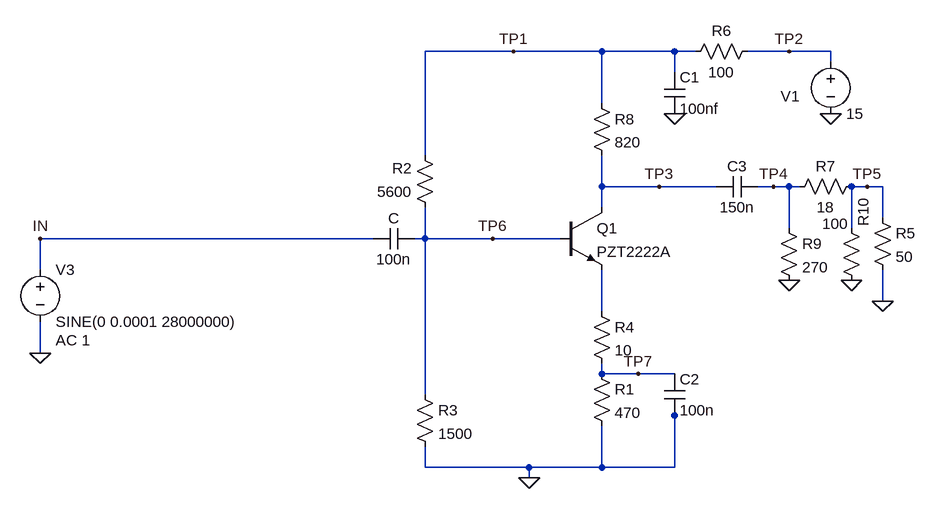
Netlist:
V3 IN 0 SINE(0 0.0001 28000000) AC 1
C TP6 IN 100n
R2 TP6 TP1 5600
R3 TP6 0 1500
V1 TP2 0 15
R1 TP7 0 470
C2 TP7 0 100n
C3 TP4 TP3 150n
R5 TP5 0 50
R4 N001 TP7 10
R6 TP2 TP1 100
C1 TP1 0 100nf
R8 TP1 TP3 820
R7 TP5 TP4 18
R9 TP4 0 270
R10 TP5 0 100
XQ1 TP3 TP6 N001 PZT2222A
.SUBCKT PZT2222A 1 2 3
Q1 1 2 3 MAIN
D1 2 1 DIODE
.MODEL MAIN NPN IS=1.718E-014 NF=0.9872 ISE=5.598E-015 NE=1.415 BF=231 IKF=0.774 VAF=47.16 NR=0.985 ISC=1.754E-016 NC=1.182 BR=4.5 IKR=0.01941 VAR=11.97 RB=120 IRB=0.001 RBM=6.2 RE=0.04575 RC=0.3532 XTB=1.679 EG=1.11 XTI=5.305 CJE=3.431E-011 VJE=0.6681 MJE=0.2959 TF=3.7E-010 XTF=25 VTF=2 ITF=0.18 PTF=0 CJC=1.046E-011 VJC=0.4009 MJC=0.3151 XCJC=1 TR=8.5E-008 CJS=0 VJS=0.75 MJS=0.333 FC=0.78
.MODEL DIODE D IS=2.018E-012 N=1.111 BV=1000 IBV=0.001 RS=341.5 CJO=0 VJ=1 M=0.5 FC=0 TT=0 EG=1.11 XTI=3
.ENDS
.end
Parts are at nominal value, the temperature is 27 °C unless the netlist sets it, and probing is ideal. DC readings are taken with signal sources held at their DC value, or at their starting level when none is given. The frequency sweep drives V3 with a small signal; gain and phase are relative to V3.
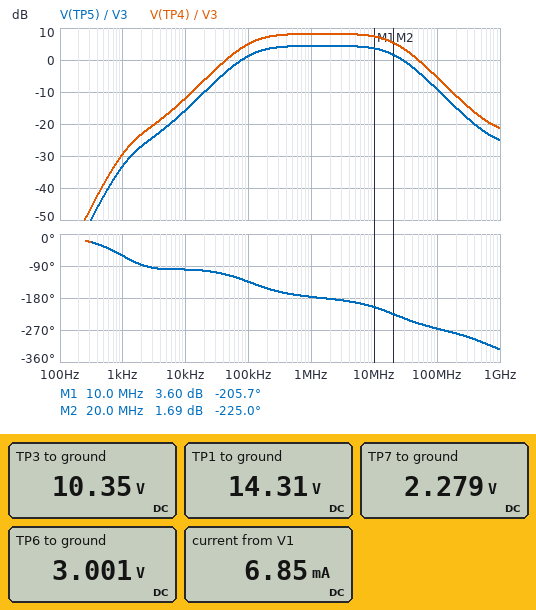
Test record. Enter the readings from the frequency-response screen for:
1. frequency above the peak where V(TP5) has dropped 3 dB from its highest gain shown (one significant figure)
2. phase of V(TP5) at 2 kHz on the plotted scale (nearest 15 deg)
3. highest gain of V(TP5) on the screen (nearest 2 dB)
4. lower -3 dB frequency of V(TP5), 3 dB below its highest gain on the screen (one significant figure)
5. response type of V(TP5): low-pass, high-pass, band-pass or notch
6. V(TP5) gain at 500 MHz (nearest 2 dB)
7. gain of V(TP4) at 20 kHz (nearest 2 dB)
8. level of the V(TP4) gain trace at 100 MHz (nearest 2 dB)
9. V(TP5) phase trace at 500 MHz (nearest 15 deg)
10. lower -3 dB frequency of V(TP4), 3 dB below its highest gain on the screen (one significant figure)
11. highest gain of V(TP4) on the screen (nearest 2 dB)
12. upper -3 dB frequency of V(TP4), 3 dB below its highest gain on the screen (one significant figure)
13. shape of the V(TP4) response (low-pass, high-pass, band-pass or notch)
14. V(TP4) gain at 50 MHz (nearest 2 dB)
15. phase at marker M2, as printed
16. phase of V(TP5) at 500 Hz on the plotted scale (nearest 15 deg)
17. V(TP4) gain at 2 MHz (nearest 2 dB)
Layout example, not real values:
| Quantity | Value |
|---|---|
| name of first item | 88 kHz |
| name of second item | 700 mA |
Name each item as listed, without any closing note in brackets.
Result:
| Quantity | Value |
|---|---|
| frequency above the peak where V(TP5) has dropped 3 dB from its highest gain shown | 20 MHz |
| phase of V(TP5) at 2 kHz on the plotted scale | -90 deg |
| highest gain of V(TP5) on the screen | 4 dB |
| lower -3 dB frequency of V(TP5), 3 dB below its highest gain on the screen | 100 kHz |
| response type of V(TP5): low-pass, high-pass, band-pass or notch | band-pass |
| V(TP5) gain at 500 MHz | -22 dB |
| gain of V(TP4) at 20 kHz | -6 dB |
| level of the V(TP4) gain trace at 100 MHz | -6 dB |
| V(TP5) phase trace at 500 MHz | -300 deg |
| lower -3 dB frequency of V(TP4), 3 dB below its highest gain on the screen | 100 kHz |
| highest gain of V(TP4) on the screen | 8 dB |
| upper -3 dB frequency of V(TP4), 3 dB below its highest gain on the screen | 20 MHz |
| shape of the V(TP4) response | band-pass |
| V(TP4) gain at 50 MHz | 0 dB |
| phase at marker M2, as printed | -225.0 deg |
| phase of V(TP5) at 500 Hz on the plotted scale | -30 deg |
| V(TP4) gain at 2 MHz | 8 dB |
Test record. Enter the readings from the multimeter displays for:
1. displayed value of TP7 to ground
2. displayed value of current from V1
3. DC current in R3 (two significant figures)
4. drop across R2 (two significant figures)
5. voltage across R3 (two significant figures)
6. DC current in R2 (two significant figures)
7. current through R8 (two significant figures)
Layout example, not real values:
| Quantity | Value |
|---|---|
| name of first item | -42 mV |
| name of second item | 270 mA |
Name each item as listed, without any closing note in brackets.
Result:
| Quantity | Value |
|---|---|
| displayed value of TP7 to ground | 2.279 V |
| displayed value of current from V1 | 6.85 mA |
| DC current in R3 | 2.0 mA |
| drop across R2 | 11 V |
| voltage across R3 | 3.0 V |
| DC current in R2 | 2.0 mA |
| current through R8 | 4.8 mA |
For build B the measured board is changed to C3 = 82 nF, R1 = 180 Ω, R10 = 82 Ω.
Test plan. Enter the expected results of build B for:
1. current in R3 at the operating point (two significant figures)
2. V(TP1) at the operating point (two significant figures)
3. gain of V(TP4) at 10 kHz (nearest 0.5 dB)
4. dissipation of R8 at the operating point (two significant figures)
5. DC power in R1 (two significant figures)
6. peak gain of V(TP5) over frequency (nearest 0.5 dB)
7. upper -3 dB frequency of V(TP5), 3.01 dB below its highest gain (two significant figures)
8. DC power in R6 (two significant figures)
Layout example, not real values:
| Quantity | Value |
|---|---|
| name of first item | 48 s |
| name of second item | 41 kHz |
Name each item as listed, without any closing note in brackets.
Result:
| Quantity | Value |
|---|---|
| current in R3 at the operating point | 1.9 mA |
| V(TP1) at the operating point | 14 V |
| gain of V(TP4) at 10 kHz | -10.5 dB |
| dissipation of R8 at the operating point | 100 mW |
| DC power in R1 | 23 mW |
| peak gain of V(TP5) over frequency | 5.5 dB |
| upper -3 dB frequency of V(TP5), 3.01 dB below its highest gain | 19 MHz |
| DC power in R6 | 17 mW |
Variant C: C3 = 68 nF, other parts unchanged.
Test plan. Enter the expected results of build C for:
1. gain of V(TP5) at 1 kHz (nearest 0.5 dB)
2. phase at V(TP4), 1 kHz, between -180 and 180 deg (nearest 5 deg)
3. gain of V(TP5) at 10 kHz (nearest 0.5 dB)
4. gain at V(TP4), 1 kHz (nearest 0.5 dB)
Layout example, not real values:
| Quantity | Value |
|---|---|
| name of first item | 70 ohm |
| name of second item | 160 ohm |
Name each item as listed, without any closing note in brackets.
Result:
| Quantity | Value |
|---|---|
| gain of V(TP5) at 1 kHz | -38.0 dB |
| phase at V(TP4), 1 kHz, between -180 and 180 deg | -40 deg |
| gain of V(TP5) at 10 kHz | -16.0 dB |
| gain at V(TP4), 1 kHz | -34.5 dB |
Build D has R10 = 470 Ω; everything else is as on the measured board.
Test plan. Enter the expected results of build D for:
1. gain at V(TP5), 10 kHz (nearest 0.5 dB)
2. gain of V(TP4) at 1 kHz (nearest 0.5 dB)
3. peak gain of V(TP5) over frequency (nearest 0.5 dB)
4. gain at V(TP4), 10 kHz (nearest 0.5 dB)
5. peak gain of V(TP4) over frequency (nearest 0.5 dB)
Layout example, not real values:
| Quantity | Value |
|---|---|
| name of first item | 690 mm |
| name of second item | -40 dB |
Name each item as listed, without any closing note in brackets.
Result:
| Quantity | Value |
|---|---|
| gain at V(TP5), 10 kHz | -13.5 dB |
| gain of V(TP4) at 1 kHz | -28.0 dB |
| peak gain of V(TP5) over frequency | 6.5 dB |
| gain at V(TP4), 10 kHz | -10.5 dB |
| peak gain of V(TP4) over frequency | 9.5 dB |
